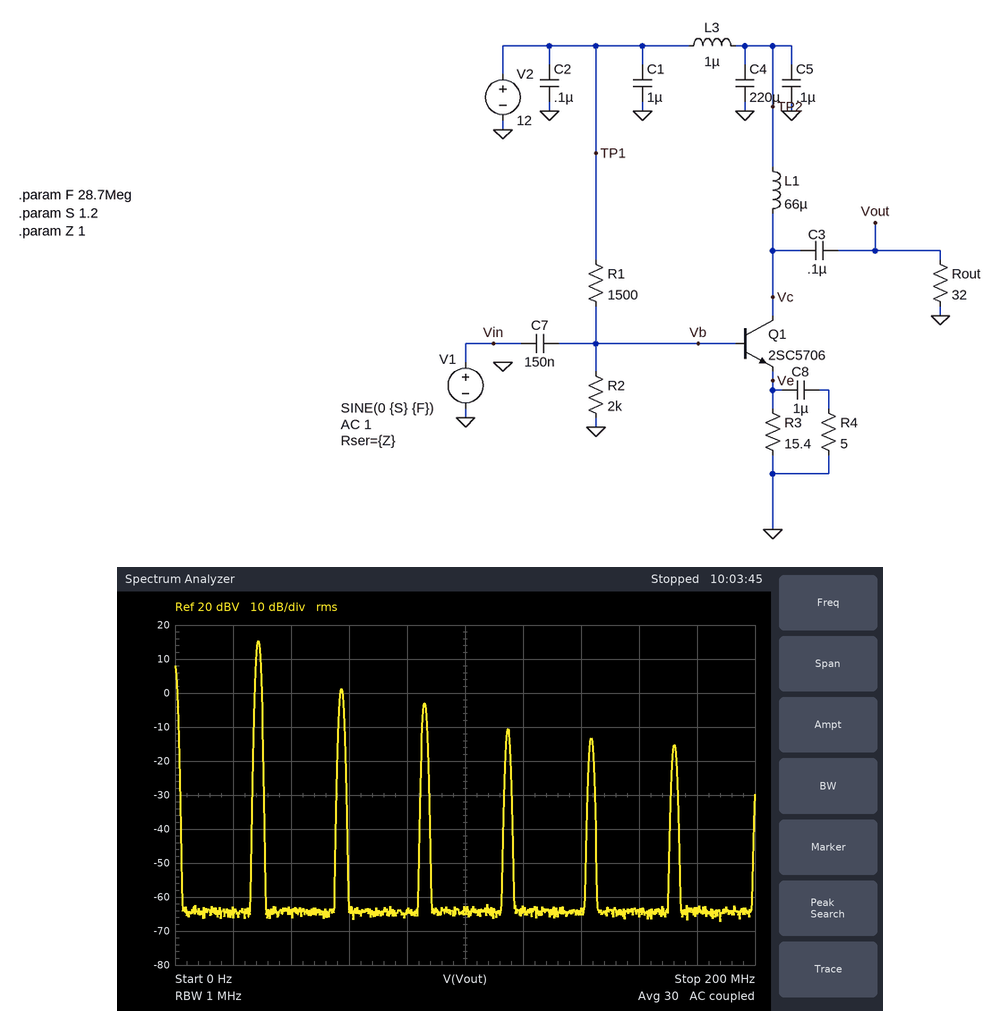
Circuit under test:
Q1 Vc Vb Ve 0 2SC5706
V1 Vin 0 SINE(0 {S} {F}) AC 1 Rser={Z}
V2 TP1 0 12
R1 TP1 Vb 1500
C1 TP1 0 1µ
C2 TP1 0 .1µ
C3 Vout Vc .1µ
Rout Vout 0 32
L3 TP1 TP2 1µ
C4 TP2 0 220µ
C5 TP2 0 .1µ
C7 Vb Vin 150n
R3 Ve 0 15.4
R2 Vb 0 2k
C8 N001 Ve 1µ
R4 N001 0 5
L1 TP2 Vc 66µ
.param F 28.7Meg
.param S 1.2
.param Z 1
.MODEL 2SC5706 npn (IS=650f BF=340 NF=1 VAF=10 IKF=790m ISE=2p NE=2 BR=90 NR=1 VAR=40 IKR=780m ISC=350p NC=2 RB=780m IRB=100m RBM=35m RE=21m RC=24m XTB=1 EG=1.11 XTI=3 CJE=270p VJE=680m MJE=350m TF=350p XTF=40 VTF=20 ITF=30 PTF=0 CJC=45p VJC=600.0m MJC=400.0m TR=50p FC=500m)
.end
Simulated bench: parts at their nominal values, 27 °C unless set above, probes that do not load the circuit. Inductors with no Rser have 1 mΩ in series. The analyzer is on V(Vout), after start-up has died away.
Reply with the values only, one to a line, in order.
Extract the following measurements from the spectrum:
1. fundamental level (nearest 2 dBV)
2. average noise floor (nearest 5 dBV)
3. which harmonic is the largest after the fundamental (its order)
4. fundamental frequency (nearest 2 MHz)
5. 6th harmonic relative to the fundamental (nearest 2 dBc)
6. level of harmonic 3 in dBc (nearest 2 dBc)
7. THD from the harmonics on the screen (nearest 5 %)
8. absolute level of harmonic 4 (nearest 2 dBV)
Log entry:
16 dBV
-65 dBV
2
28 MHz
-30 dBc
-18 dBc
25 %
-10 dBV
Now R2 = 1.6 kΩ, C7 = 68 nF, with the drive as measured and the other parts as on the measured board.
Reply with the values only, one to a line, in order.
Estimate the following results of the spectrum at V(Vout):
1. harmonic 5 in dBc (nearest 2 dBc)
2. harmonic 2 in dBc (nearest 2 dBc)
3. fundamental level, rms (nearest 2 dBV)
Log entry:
-36 dBc
-18 dBc
16 dBV
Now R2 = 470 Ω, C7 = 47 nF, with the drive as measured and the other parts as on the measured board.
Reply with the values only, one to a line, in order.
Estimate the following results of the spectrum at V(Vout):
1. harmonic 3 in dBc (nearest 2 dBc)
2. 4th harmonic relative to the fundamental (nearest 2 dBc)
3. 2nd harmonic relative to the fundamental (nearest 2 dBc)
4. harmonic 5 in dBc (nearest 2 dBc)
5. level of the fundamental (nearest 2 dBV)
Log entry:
-20 dBc
-32 dBc
-12 dBc
-30 dBc
14 dBV
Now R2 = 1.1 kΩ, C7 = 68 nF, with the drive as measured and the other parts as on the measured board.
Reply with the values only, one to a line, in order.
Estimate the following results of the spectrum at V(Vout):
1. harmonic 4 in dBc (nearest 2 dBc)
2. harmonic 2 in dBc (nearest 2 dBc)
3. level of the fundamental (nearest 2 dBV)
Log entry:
-30 dBc
-26 dBc
16 dBV
